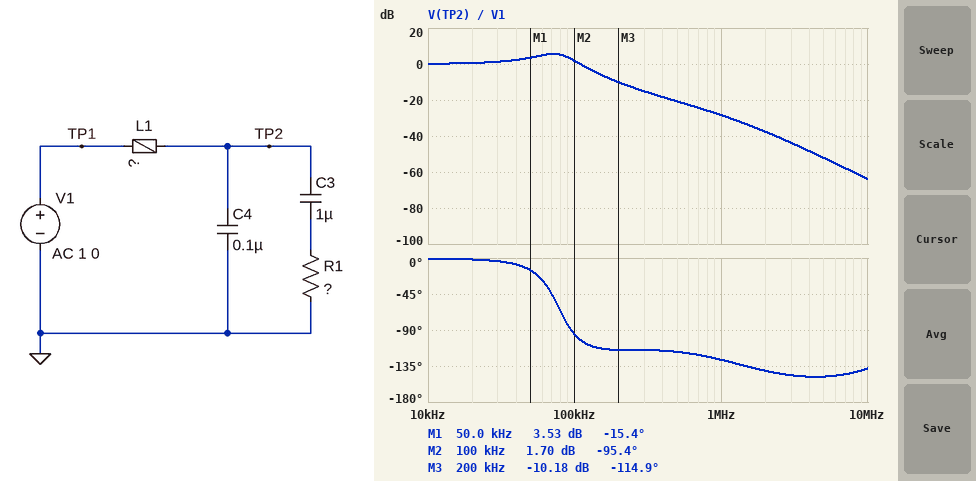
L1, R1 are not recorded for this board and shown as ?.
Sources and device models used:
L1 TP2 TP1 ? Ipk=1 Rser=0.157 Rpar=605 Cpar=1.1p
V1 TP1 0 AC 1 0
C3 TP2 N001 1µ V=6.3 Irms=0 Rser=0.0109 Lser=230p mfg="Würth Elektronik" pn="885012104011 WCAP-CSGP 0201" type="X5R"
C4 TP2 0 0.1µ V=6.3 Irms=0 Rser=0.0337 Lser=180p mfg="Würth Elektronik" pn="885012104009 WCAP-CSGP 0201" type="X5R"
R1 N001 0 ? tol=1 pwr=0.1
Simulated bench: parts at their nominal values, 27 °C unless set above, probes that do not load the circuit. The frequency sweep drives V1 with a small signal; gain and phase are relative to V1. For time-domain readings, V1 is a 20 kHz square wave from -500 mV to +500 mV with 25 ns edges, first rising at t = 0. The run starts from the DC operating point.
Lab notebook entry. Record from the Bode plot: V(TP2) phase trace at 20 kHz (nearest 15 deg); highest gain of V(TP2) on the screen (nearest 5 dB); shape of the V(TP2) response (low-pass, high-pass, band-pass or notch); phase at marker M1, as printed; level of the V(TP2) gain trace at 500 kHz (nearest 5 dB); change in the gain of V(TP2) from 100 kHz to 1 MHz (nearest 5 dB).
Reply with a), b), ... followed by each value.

a) 0 deg
b) 5 dB
c) low-pass
d) -15.4 deg
e) -20 dB
f) -30 dB
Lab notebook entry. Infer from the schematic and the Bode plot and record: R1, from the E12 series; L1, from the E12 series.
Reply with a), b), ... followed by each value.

a) 1.2 Ω
b) 3.9 µH
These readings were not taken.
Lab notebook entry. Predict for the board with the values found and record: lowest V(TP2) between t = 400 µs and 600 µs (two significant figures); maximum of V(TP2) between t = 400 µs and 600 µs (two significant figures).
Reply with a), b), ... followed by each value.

a) -930 mV
b) 930 mV
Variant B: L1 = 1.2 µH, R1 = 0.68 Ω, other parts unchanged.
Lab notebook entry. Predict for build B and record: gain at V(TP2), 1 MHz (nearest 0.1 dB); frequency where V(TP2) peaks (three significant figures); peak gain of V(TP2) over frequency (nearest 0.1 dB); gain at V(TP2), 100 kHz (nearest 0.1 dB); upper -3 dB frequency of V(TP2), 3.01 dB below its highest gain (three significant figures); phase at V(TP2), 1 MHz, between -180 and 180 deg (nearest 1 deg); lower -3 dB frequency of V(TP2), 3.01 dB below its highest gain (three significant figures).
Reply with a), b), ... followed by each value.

a) -21.7 dB
b) 127 kHz
c) 4.7 dB
d) 3.8 dB
e) 175 kHz
f) -118 deg
g) 63.9 kHz
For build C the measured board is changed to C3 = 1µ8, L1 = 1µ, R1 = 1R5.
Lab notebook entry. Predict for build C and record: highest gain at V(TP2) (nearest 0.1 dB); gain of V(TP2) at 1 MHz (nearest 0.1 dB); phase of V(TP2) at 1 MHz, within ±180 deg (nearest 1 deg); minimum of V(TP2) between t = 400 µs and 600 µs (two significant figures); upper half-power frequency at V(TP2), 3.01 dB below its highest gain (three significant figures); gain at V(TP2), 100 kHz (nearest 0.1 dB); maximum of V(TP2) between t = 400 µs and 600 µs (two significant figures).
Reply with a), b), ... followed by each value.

a) 0.7 dB
b) -14.5 dB
c) -125 deg
d) -580 mV
e) 285 kHz
f) 0.6 dB
g) 580 mV
